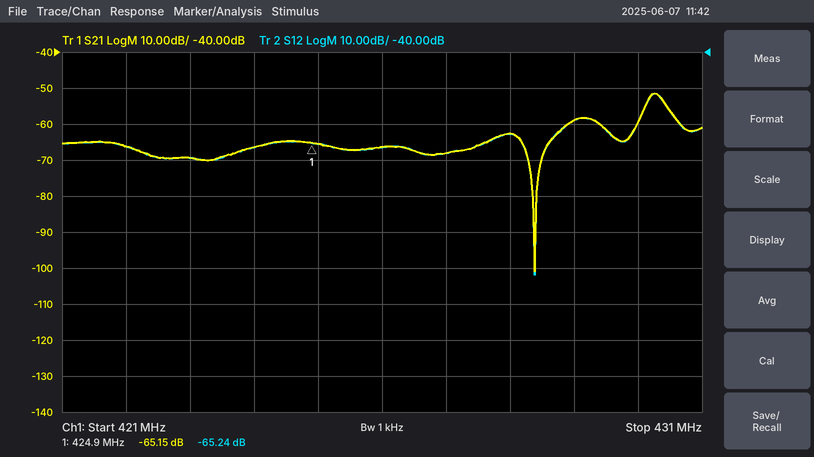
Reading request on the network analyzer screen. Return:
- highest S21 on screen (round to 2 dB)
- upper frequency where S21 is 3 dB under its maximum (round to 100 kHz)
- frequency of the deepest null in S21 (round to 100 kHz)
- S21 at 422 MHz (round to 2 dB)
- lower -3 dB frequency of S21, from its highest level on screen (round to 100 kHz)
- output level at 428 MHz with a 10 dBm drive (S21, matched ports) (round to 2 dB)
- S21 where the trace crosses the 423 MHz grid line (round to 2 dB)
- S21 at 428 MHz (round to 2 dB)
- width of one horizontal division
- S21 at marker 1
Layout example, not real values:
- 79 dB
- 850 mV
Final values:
- -52 dB
- 430.4 MHz
- 428.4 MHz
- -66 dB
- 430.1 MHz
- -52 dBm
- -70 dB
- -62 dB
- 1 MHz
- -65.15 dB
